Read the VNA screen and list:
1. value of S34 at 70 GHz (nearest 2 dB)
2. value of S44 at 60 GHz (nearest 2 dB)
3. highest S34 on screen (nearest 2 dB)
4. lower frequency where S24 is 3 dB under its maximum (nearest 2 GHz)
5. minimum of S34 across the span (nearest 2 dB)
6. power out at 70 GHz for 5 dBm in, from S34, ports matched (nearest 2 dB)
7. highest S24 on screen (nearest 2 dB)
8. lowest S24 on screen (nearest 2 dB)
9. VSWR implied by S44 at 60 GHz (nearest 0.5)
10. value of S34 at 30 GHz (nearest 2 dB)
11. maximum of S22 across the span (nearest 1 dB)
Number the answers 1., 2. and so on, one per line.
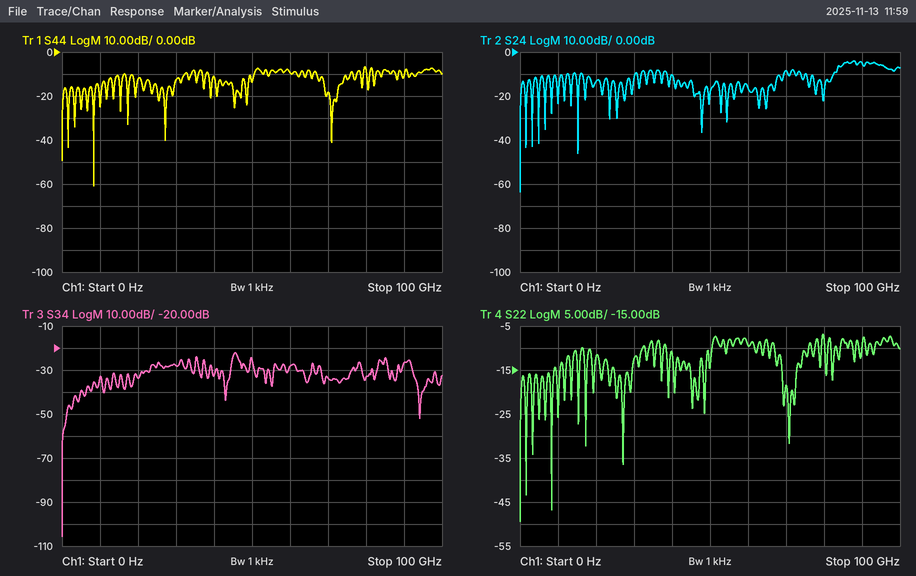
1. -34 dB
2. -10 dB
3. -22 dB
4. 84 GHz
5. -106 dB
6. -28 dBm
7. -4 dB
8. -64 dB
9. 2.0
10. -28 dB
11. -7 dB
